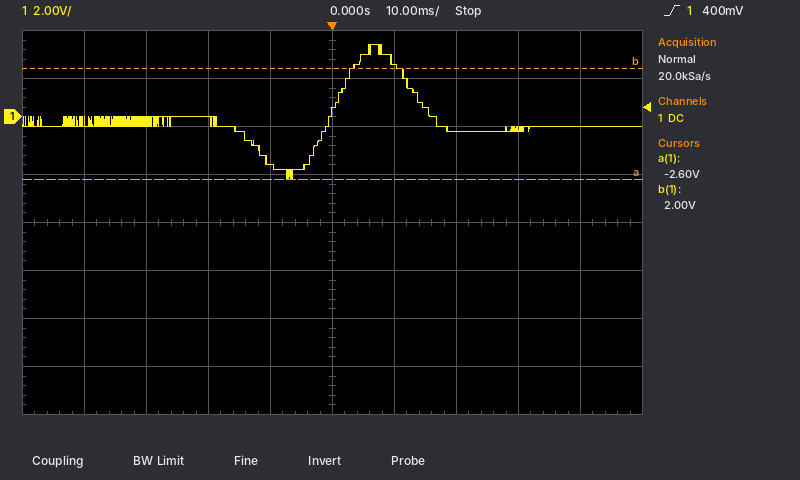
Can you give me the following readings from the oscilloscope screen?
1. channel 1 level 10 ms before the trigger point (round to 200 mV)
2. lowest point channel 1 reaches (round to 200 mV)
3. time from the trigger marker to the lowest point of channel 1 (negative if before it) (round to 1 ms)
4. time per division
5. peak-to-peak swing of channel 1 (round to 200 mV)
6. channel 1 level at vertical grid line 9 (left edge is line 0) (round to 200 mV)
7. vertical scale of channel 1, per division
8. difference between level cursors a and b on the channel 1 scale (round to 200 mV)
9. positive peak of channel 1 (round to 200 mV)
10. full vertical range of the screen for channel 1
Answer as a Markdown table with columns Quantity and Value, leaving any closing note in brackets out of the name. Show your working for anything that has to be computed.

| Quantity | Value |
|---|---|
| channel 1 level 10 ms before the trigger point | -2.0 V |
| lowest point channel 1 reaches | -2.6 V |
| time from the trigger marker to the lowest point of channel 1 (negative if before it) | -7 ms |
| time per division | 10 ms |
| peak-to-peak swing of channel 1 | 3.0 V − (-2.6 V) = 5.6 V |
| channel 1 level at vertical grid line 9 (left edge is line 0) | -400 mV |
| vertical scale of channel 1, per division | 2 V |
| difference between level cursors a and b on the channel 1 scale | 4.6 V |
| positive peak of channel 1 | 3.0 V |
| full vertical range of the screen for channel 1 | 16 V |
